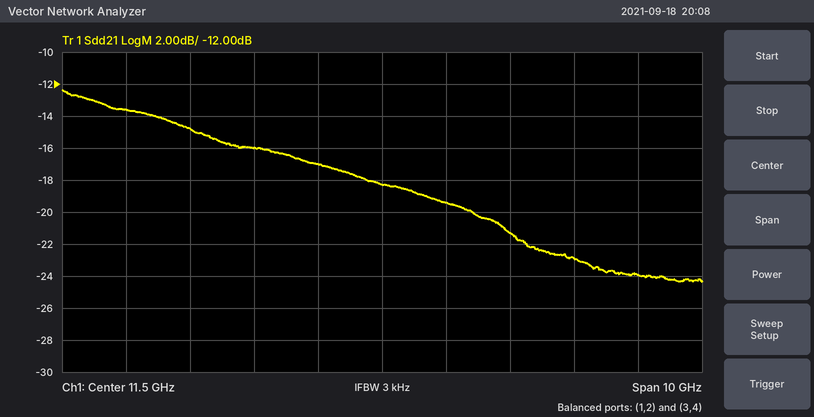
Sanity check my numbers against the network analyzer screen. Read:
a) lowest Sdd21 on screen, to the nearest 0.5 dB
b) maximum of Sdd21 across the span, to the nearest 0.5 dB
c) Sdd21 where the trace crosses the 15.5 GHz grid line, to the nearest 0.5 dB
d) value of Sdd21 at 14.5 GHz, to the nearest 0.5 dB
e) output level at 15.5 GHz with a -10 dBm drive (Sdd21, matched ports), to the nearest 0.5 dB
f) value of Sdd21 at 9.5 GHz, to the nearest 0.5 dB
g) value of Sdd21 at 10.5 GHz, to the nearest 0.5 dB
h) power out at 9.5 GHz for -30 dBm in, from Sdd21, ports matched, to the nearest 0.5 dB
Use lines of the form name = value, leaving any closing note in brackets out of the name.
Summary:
lowest Sdd21 on screen, to the nearest 0.5 dB = -24.5 dB
maximum of Sdd21 across the span, to the nearest 0.5 dB = -12.5 dB
Sdd21 where the trace crosses the 15.5 GHz grid line, to the nearest 0.5 dB = -24.0 dB
value of Sdd21 at 14.5 GHz, to the nearest 0.5 dB = -23.0 dB
output level at 15.5 GHz with a -10 dBm drive (Sdd21, matched ports), to the nearest 0.5 dB = -34.0 dBm
value of Sdd21 at 9.5 GHz, to the nearest 0.5 dB = -16.0 dB
value of Sdd21 at 10.5 GHz, to the nearest 0.5 dB = -17.0 dB
power out at 9.5 GHz for -30 dBm in, from Sdd21, ports matched, to the nearest 0.5 dB = -46.0 dBm
